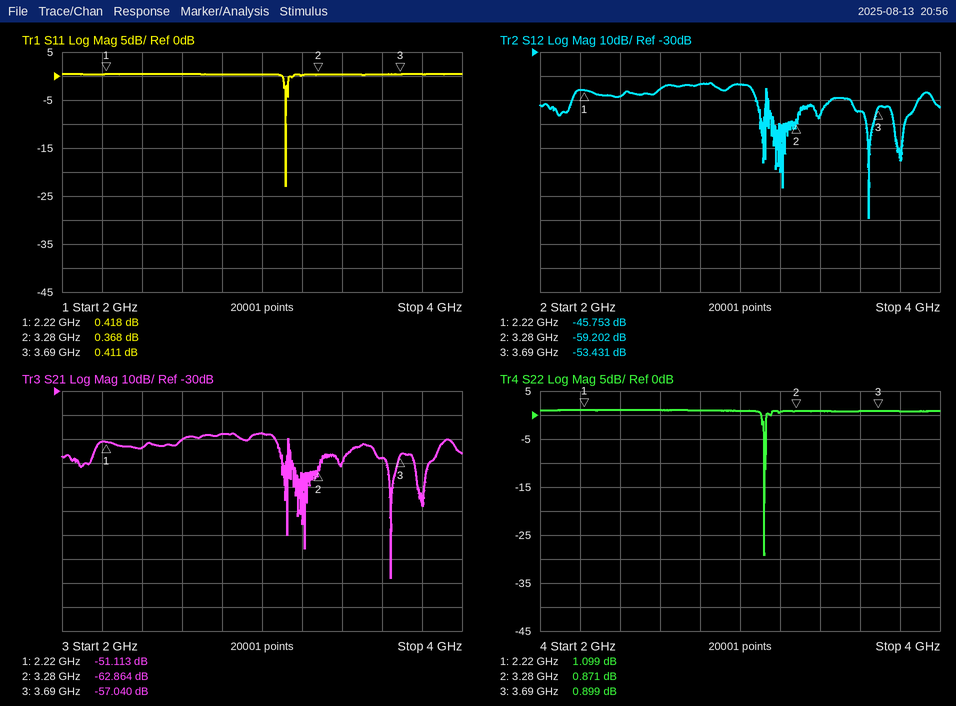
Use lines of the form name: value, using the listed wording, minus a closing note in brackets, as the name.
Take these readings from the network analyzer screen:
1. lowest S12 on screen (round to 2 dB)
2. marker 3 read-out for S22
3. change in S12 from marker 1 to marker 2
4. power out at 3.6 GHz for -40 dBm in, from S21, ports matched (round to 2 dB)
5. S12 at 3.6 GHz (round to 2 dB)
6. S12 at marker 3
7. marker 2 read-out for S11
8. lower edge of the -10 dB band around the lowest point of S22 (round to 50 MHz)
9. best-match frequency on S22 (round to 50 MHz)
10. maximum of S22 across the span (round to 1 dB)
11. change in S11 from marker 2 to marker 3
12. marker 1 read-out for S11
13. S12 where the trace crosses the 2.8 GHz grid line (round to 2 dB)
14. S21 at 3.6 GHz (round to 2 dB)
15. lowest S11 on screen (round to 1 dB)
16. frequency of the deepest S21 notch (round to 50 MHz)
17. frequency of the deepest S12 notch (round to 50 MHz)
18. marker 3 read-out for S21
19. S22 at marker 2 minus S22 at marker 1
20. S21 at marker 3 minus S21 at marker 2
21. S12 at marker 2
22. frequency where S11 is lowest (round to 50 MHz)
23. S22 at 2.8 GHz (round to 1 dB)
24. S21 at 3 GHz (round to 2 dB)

lowest S12 on screen: -100 dB
marker 3 read-out for S22: 0.899 dB
change in S12 from marker 1 to marker 2: -13.449 dB
power out at 3.6 GHz for -40 dBm in, from S21, ports matched: -98 dBm
S12 at 3.6 GHz: -54 dB
S12 at marker 3: -53.431 dB
marker 2 read-out for S11: 0.368 dB
lower edge of the -10 dB band around the lowest point of S22: 3.10 GHz
best-match frequency on S22: 3.10 GHz
maximum of S22 across the span: 1 dB
change in S11 from marker 2 to marker 3: 0.043 dB
marker 1 read-out for S11: 0.418 dB
S12 where the trace crosses the 2.8 GHz grid line: -44 dB
S21 at 3.6 GHz: -58 dB
lowest S11 on screen: -23 dB
frequency of the deepest S21 notch: 3.65 GHz
frequency of the deepest S12 notch: 3.65 GHz
marker 3 read-out for S21: -57.040 dB
S22 at marker 2 minus S22 at marker 1: -0.228 dB
S21 at marker 3 minus S21 at marker 2: 5.824 dB
S12 at marker 2: -59.202 dB
frequency where S11 is lowest: 3.10 GHz
S22 at 2.8 GHz: 1 dB
S21 at 3 GHz: -48 dB
